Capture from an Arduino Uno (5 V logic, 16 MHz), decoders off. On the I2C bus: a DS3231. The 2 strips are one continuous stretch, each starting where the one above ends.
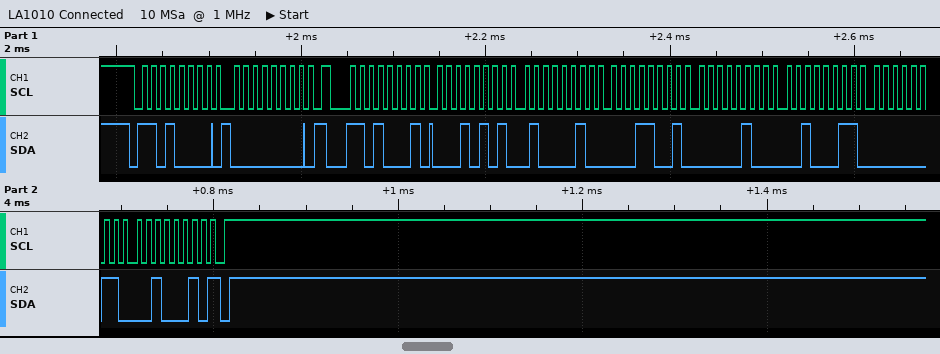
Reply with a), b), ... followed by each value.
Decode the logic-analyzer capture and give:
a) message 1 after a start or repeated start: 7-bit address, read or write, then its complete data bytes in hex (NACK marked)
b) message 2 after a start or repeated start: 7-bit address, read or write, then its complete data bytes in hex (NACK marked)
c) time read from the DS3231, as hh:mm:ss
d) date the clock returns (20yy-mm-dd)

a) 0x68 write: 00
b) 0x68 read: 15 42 19 04 23 03 22 NACK
c) 19:42:15
d) 2022-03-23
